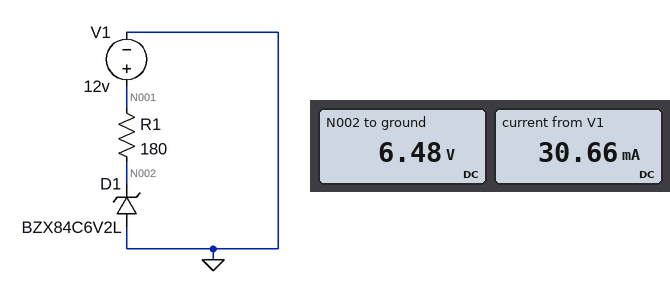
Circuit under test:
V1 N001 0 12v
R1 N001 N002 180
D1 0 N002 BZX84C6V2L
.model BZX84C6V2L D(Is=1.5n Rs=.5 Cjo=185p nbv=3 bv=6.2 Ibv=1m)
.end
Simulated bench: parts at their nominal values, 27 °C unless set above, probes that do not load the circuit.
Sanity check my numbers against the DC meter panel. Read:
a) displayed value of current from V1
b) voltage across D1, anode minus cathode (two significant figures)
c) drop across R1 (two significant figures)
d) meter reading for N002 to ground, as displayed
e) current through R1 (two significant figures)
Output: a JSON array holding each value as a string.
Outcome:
["30.66 mA", "-6.5 V", "5.5 V", "6.48 V", "31 mA"]
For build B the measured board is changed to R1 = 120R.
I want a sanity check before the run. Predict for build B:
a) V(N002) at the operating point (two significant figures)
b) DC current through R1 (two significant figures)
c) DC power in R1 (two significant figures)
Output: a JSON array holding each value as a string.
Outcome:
["6.5 V", "46 mA", "250 mW"]
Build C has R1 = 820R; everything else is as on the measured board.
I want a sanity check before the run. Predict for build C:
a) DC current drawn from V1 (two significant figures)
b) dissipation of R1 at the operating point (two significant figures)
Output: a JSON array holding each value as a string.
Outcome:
["6.9 mA", "39 mW"]
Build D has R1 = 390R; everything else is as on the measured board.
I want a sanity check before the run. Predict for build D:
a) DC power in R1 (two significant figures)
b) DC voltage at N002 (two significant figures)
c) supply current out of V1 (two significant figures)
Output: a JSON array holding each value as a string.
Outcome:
["80 mW", "6.4 V", "14 mA"]
